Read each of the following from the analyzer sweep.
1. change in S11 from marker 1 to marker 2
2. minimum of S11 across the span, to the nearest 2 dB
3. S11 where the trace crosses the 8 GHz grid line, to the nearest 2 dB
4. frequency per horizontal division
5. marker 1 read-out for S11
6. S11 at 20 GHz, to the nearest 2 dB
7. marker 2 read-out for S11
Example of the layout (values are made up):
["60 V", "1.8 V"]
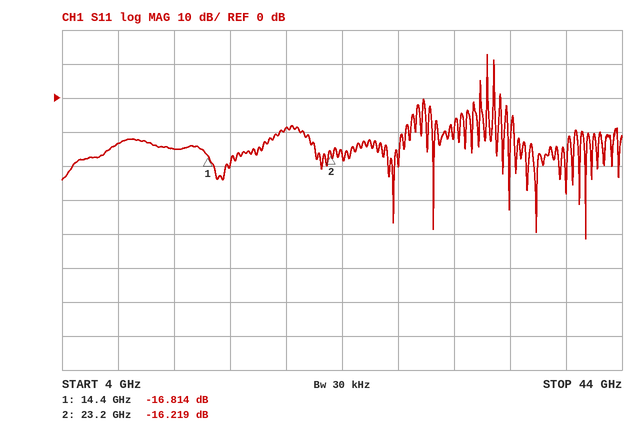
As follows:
["0.595 dB", "-42 dB", "-14 dB", "4 GHz", "-16.814 dB", "-8 dB", "-16.219 dB"]
